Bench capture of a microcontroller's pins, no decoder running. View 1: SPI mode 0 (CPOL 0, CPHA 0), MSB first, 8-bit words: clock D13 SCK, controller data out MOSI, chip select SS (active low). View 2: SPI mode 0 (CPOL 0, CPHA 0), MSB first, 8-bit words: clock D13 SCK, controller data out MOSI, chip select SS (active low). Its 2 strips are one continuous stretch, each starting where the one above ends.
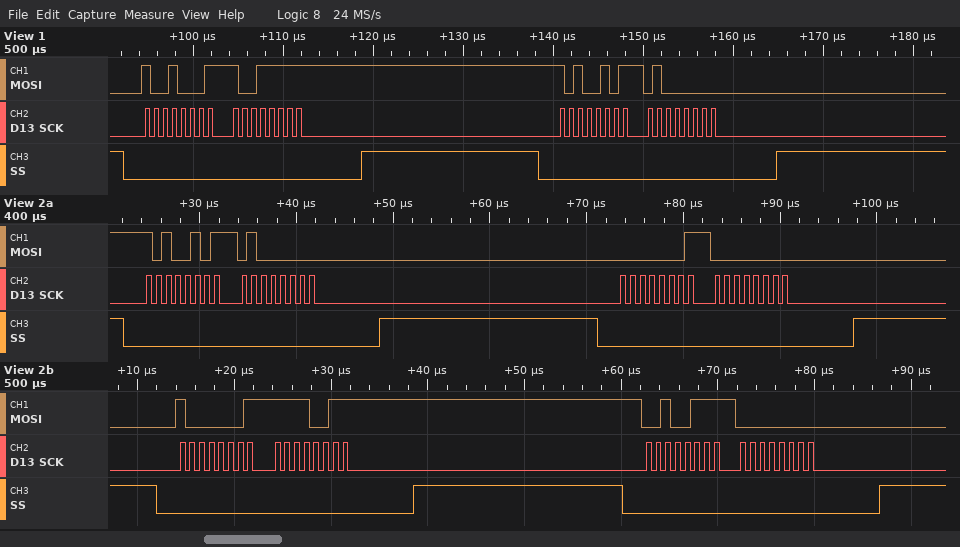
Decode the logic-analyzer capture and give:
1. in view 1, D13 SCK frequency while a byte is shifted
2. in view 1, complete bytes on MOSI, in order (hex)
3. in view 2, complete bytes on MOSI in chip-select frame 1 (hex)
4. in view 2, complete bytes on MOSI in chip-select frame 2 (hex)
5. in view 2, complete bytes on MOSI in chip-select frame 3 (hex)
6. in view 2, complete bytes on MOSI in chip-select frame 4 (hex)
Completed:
1 MHz
91 9F A5 40
A5 40
01 00
81 F3
27 00
